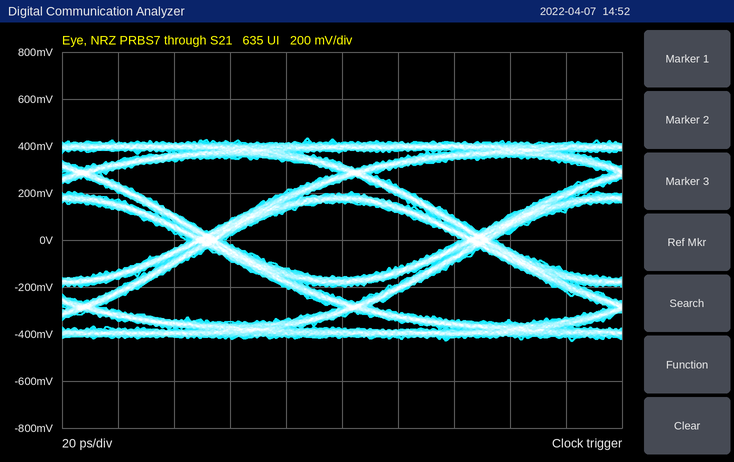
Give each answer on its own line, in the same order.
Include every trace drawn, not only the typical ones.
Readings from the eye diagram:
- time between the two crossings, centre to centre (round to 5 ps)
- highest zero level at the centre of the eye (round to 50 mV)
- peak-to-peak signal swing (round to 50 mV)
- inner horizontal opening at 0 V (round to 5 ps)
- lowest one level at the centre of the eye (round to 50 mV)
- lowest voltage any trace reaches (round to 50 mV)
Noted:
95 ps
-150 mV
850 mV
85 ps
150 mV
-450 mV
